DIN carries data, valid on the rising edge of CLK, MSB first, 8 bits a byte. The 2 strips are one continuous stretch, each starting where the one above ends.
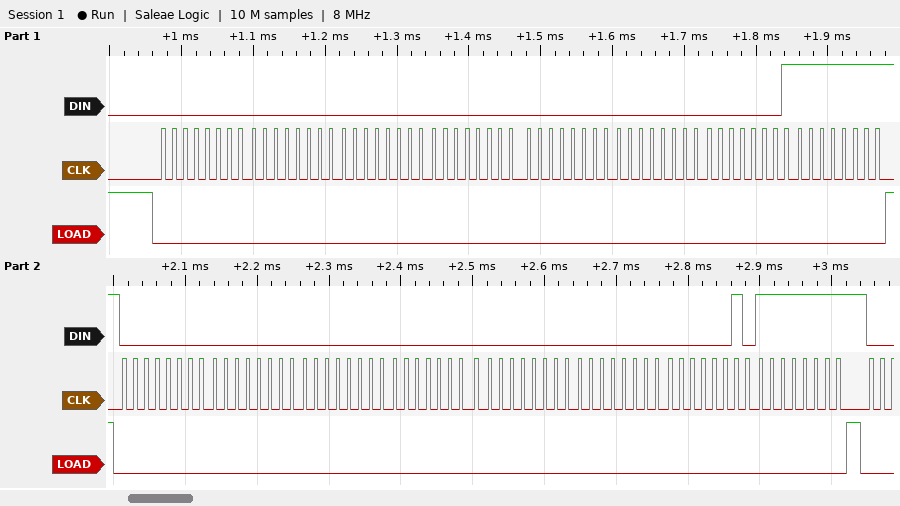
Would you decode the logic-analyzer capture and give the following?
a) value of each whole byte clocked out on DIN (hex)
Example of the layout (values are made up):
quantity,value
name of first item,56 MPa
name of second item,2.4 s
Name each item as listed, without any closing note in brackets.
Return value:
quantity,value
value of each whole byte clocked out on DIN,0x00 0x00 0x00 0x00 0x00 0x00 0x01 0xFF 0x00 0x00 0x00 0x00 0x00 0x00 0x02 0xFF
